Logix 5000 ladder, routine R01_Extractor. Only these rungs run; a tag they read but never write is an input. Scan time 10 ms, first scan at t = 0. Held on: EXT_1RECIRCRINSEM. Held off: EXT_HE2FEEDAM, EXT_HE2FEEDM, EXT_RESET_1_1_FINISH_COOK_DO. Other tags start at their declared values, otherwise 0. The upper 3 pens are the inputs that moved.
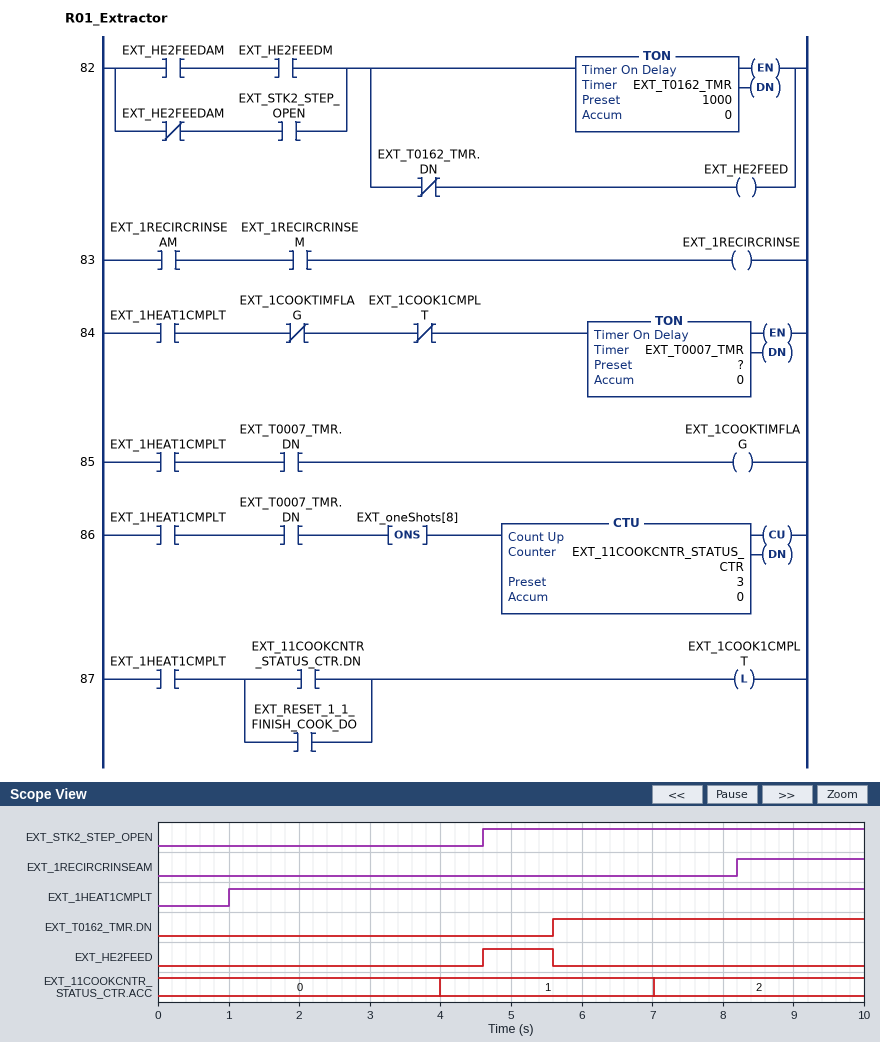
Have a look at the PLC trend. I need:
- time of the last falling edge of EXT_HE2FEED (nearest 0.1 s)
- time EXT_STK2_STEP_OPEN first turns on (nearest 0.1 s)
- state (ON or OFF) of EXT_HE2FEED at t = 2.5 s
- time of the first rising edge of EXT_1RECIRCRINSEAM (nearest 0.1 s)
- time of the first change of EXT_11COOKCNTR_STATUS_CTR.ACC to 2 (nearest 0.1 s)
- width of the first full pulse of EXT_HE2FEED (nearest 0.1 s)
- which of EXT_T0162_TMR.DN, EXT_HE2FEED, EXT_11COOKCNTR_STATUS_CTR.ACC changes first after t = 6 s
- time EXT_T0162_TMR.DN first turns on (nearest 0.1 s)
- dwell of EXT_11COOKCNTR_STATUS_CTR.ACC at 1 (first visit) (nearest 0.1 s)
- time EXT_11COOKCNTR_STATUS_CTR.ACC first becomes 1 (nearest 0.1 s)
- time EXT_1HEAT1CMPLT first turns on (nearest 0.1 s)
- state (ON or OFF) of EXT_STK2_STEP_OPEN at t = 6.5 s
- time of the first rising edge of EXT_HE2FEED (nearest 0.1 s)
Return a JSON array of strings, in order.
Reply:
["5.6 s", "4.6 s", "OFF", "8.2 s", "7.0 s", "1.0 s", "EXT_11COOKCNTR_STATUS_CTR.ACC", "5.6 s", "3.0 s", "4.0 s", "1.0 s", "ON", "4.6 s"]
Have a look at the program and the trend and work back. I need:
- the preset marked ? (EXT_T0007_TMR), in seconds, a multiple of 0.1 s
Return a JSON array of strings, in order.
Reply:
["3.0 s"]
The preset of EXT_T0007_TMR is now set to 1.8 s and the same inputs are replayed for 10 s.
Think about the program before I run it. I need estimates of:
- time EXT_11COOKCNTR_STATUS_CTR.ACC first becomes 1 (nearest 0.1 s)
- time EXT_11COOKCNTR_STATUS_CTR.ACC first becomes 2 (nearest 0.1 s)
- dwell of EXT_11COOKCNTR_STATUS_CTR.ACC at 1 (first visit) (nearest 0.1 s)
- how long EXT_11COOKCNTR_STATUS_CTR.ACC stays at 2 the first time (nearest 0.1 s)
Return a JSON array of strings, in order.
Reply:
["2.8 s", "4.6 s", "1.8 s", "1.8 s"]
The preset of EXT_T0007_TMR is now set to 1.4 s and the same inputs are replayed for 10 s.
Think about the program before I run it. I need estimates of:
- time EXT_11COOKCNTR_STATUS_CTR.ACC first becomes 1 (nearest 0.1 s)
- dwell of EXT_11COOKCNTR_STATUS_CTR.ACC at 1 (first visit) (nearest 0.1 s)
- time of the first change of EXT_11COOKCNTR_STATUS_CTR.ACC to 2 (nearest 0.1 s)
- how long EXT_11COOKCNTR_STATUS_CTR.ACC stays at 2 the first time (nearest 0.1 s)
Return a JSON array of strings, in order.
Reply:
["2.4 s", "1.4 s", "3.8 s", "1.4 s"]
